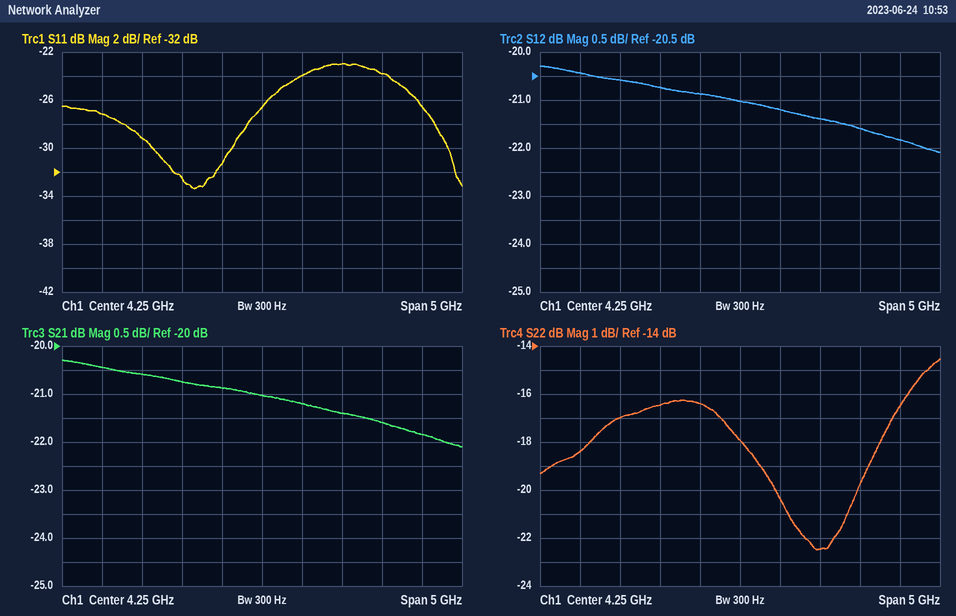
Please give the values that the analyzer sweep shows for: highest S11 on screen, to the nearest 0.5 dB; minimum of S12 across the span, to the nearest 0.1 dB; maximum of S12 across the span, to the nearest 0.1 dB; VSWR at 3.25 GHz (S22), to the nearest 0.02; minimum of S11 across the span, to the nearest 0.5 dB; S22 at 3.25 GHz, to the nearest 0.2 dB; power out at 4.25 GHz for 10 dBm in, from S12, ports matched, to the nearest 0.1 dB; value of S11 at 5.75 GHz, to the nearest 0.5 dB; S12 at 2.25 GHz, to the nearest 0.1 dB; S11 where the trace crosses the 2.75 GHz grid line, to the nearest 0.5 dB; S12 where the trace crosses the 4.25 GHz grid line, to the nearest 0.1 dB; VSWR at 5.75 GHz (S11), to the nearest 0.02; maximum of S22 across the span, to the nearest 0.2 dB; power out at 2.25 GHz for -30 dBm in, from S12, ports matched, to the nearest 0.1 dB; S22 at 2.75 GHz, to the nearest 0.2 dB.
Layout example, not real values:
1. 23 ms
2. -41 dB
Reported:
1. -23.0 dB
2. -22.1 dB
3. -20.3 dB
4. 1.36
5. -33.5 dB
6. -16.4 dB
7. -11.0 dBm
8. -24.0 dB
9. -20.4 dB
10. -29.0 dB
11. -21.0 dB
12. 1.14
13. -14.6 dB
14. -50.4 dBm
15. -17.0 dB
